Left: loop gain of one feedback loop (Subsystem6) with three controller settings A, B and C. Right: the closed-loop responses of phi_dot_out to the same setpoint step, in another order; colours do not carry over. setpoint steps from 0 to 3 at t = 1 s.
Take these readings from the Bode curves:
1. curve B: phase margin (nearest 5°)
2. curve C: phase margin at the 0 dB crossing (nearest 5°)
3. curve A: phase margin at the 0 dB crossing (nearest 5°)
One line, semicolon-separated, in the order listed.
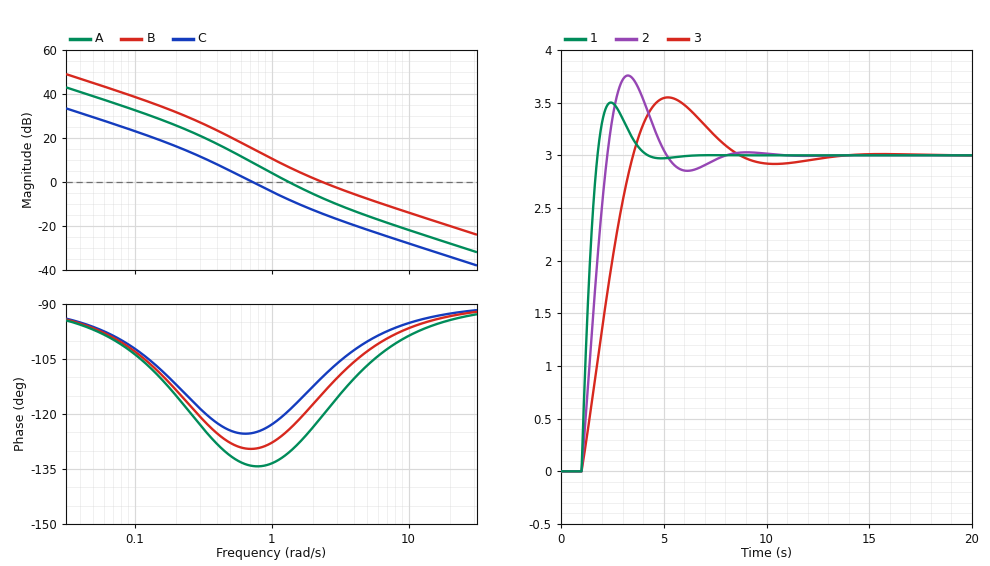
65°; 55°; 50°
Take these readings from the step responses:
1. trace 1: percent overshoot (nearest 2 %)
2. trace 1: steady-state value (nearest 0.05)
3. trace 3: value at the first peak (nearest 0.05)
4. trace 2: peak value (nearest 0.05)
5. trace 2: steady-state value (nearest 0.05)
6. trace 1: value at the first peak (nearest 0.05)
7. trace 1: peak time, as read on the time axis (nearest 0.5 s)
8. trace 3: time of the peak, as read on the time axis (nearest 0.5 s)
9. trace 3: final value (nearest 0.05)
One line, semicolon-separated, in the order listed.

16 %; 3.00; 3.55; 3.75; 3.00; 3.50; 2.5 s; 5.0 s; 3.00
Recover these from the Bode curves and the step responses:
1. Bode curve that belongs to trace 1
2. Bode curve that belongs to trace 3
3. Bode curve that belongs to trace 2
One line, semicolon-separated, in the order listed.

B; C; A
